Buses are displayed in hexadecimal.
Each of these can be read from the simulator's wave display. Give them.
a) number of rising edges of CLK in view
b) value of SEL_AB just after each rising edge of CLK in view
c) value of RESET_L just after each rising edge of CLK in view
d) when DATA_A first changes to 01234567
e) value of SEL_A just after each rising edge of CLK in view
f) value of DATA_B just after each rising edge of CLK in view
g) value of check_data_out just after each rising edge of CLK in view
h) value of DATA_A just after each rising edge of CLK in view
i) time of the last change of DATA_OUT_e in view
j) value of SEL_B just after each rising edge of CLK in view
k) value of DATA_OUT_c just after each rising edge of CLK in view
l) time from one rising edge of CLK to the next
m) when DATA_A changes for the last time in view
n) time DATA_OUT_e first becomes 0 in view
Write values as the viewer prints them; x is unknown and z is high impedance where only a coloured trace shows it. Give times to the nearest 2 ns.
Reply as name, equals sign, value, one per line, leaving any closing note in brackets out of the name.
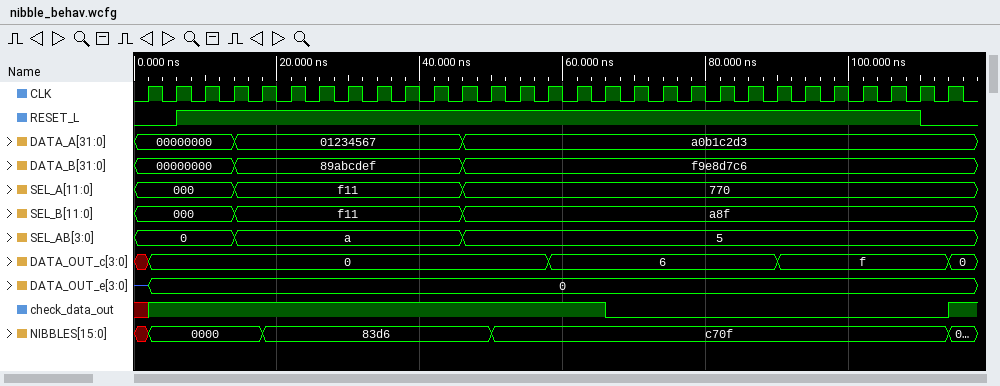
number of rising edges of CLK in view = 29
value of SEL_AB just after each rising edge of CLK in view = 0, 0, 0, a, a, a, a, a, a, a, a, 5, 5, 5, 5, 5, 5, 5, 5, 5, 5, 5, 5, 5, 5, 5, 5, 5, 5
value of RESET_L just after each rising edge of CLK in view = 0 1 1 1 1 1 1 1 1 1 1 1 1 1 1 1 1 1 1 1 1 1 1 1 1 1 1 0 0
when DATA_A first changes to 01234567 = 14 ns
value of SEL_A just after each rising edge of CLK in view = 000, 000, 000, f11, f11, f11, f11, f11, f11, f11, f11, 770, 770, 770, 770, 770, 770, 770, 770, 770, 770, 770, 770, 770, 770, 770, 770, 770, 770
value of DATA_B just after each rising edge of CLK in view = 00000000, 00000000, 00000000, 89abcdef, 89abcdef, 89abcdef, 89abcdef, 89abcdef, 89abcdef, 89abcdef, 89abcdef, f9e8d7c6, f9e8d7c6, f9e8d7c6, f9e8d7c6, f9e8d7c6, f9e8d7c6, f9e8d7c6, f9e8d7c6, f9e8d7c6, f9e8d7c6, f9e8d7c6, f9e8d7c6, f9e8d7c6, f9e8d7c6, f9e8d7c6, f9e8d7c6, f9e8d7c6, f9e8d7c6
value of check_data_out just after each rising edge of CLK in view = 1 1 1 1 1 1 1 1 1 1 1 1 1 1 1 1 0 0 0 0 0 0 0 0 0 0 0 0 1
value of DATA_A just after each rising edge of CLK in view = 00000000, 00000000, 00000000, 01234567, 01234567, 01234567, 01234567, 01234567, 01234567, 01234567, 01234567, a0b1c2d3, a0b1c2d3, a0b1c2d3, a0b1c2d3, a0b1c2d3, a0b1c2d3, a0b1c2d3, a0b1c2d3, a0b1c2d3, a0b1c2d3, a0b1c2d3, a0b1c2d3, a0b1c2d3, a0b1c2d3, a0b1c2d3, a0b1c2d3, a0b1c2d3, a0b1c2d3
time of the last change of DATA_OUT_e in view = 2 ns
value of SEL_B just after each rising edge of CLK in view = 000, 000, 000, f11, f11, f11, f11, f11, f11, f11, f11, a8f, a8f, a8f, a8f, a8f, a8f, a8f, a8f, a8f, a8f, a8f, a8f, a8f, a8f, a8f, a8f, a8f, a8f
value of DATA_OUT_c just after each rising edge of CLK in view = 0, 0, 0, 0, 0, 0, 0, 0, 0, 0, 0, 0, 0, 0, 6, 6, 6, 6, 6, 6, 6, 6, f, f, f, f, f, f, 0
time from one rising edge of CLK to the next = 4 ns
when DATA_A changes for the last time in view = 46 ns
time DATA_OUT_e first becomes 0 in view = 2 ns
